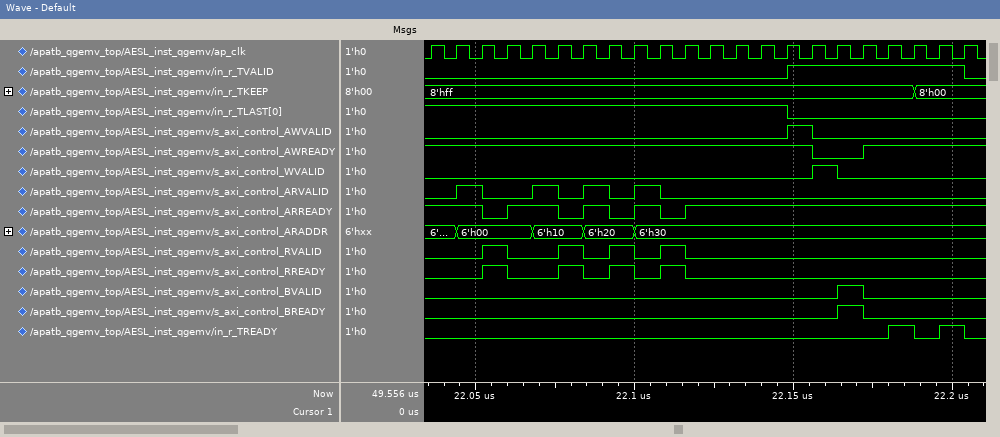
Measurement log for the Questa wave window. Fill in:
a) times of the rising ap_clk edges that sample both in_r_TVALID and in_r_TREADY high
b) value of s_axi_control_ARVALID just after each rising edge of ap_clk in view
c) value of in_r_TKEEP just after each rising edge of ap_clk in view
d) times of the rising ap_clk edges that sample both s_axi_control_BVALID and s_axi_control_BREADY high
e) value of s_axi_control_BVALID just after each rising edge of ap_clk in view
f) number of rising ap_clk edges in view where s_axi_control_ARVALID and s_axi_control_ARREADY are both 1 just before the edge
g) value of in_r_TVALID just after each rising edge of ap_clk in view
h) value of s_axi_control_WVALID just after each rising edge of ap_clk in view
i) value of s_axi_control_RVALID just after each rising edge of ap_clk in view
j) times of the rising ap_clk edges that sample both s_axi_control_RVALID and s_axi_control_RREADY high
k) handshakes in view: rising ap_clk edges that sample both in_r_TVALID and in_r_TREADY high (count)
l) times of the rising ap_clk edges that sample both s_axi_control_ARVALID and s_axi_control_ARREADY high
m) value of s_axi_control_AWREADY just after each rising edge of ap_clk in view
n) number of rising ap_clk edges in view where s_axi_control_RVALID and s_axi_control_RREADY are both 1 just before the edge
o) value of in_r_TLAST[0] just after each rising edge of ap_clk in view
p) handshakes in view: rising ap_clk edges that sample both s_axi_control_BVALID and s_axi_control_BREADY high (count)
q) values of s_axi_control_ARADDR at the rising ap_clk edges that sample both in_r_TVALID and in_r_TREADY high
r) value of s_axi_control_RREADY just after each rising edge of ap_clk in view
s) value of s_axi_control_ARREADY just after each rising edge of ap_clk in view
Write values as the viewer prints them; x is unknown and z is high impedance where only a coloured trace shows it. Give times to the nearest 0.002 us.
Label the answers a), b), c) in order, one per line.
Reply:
a) 22.188 us, 22.204 us
b) 0 1 0 0 1 0 1 0 1 0 0 0 0 0 0 0 0 0 0 0 0 0
c) 8'hff, 8'hff, 8'hff, 8'hff, 8'hff, 8'hff, 8'hff, 8'hff, 8'hff, 8'hff, 8'hff, 8'hff, 8'hff, 8'hff, 8'hff, 8'hff, 8'hff, 8'hff, 8'hff, 8'h00, 8'h00, 8'h00
d) 22.172 us
e) 0 0 0 0 0 0 0 0 0 0 0 0 0 0 0 0 1 0 0 0 0 0
f) 4
g) 0 0 0 0 0 0 0 0 0 0 0 0 0 0 1 1 1 1 1 1 1 0
h) 0 0 0 0 0 0 0 0 0 0 0 0 0 0 0 1 0 0 0 0 0 0
i) 0 0 1 0 0 1 0 1 0 1 0 0 0 0 0 0 0 0 0 0 0 0
j) 22.06 us, 22.084 us, 22.1 us, 22.116 us
k) 2
l) 22.052 us, 22.076 us, 22.092 us, 22.108 us
m) 1 1 1 1 1 1 1 1 1 1 1 1 1 1 1 0 0 1 1 1 1 1
n) 4
o) 1 1 1 1 1 1 1 1 1 1 1 1 1 1 0 0 0 0 0 0 0 0
p) 1
q) 6'h30, 6'h30
r) 0 0 1 0 0 1 0 1 0 1 0 0 0 0 0 0 0 0 0 0 0 0
s) 1 1 0 1 1 0 1 0 1 0 1 1 1 1 1 1 1 1 1 1 1 1
